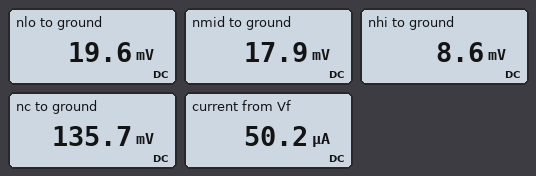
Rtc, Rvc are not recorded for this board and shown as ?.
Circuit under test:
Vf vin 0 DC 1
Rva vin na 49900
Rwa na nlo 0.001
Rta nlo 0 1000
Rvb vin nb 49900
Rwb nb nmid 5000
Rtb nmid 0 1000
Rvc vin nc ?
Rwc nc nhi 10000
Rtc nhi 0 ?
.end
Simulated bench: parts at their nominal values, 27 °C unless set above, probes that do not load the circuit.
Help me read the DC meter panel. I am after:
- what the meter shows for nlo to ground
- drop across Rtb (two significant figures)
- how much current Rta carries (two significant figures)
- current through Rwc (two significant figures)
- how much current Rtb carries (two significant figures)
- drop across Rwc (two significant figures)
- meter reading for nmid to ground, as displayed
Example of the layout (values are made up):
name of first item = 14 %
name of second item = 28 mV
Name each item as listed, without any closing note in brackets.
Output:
what the meter shows for nlo to ground = 19.6 mV
drop across Rtb = 18 mV
how much current Rta carries = 20 µA
current through Rwc = 13 µA
how much current Rtb carries = 18 µA
drop across Rwc = 130 mV
meter reading for nmid to ground, as displayed = 17.9 mV
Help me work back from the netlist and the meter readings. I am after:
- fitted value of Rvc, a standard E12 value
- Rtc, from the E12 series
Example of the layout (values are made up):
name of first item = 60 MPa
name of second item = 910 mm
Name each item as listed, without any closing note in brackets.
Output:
fitted value of Rvc, a standard E12 value = 68 kΩ
Rtc, from the E12 series = 680 Ω
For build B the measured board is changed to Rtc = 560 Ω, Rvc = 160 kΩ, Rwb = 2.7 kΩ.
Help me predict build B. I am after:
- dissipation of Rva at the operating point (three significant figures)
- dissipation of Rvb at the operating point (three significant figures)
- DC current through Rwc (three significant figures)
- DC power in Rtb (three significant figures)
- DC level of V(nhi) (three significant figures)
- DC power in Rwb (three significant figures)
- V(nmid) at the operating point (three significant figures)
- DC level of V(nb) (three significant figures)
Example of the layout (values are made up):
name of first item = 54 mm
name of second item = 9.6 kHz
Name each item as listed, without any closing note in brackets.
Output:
dissipation of Rva at the operating point = 19.3 µW
dissipation of Rvb at the operating point = 17.4 µW
DC current through Rwc = 5.86 µA
DC power in Rtb = 348 nW
DC level of V(nhi) = 3.28 mV
DC power in Rwb = 940 nW
V(nmid) at the operating point = 18.7 mV
DC level of V(nb) = 69.0 mV
